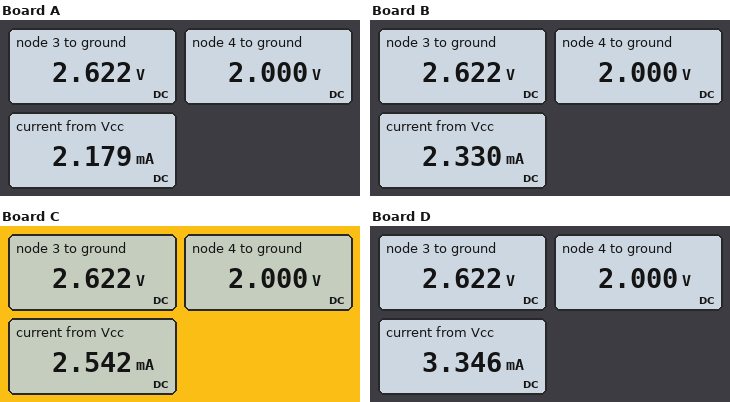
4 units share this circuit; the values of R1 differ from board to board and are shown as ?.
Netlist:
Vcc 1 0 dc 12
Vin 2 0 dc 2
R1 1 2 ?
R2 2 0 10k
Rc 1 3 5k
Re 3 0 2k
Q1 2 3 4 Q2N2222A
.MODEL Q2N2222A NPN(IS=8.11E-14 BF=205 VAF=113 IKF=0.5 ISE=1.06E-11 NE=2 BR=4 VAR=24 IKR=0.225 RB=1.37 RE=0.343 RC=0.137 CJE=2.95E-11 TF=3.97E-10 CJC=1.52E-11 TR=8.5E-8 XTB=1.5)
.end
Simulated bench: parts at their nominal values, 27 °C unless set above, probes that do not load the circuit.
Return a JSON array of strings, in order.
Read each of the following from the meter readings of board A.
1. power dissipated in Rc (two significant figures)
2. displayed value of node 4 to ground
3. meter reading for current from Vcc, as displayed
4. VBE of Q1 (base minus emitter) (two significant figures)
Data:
["18 mW", "2.000 V", "2.179 mA", "620 mV"]
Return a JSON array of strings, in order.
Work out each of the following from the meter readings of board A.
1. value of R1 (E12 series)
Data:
["33 kΩ"]
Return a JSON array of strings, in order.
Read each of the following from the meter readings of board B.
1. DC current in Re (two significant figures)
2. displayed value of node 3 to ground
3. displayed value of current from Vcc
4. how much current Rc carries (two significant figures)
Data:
["1.3 mA", "2.622 V", "2.330 mA", "1.9 mA"]
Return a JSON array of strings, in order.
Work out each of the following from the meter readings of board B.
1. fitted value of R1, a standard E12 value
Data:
["22 kΩ"]
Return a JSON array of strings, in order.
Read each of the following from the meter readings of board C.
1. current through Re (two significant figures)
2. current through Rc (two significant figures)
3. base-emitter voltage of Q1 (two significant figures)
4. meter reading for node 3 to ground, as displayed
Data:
["1.3 mA", "1.9 mA", "620 mV", "2.622 V"]
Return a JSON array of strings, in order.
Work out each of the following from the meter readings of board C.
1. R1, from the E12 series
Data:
["15 kΩ"]
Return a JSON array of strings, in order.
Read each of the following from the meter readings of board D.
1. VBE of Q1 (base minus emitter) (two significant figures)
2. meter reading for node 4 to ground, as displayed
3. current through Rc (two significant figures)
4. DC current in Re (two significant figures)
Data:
["620 mV", "2.000 V", "1.9 mA", "1.3 mA"]
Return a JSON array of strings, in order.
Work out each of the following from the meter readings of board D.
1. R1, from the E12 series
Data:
["6.8 kΩ"]
